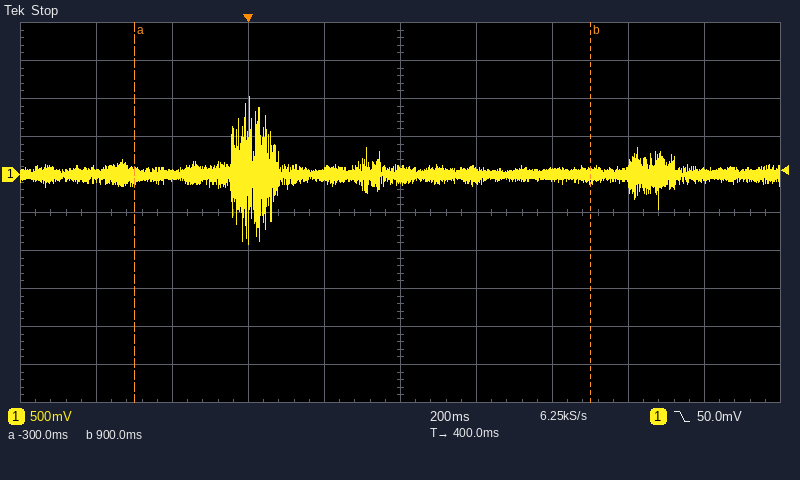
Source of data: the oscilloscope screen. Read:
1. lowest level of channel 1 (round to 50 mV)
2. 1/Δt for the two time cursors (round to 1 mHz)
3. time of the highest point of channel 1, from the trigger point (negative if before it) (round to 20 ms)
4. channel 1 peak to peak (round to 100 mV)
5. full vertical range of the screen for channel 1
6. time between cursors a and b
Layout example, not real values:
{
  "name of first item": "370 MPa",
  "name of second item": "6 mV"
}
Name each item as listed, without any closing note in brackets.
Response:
{
  "lowest level of channel 1": "-900 mV",
  "1/Δt for the two time cursors": "833 mHz",
  "time of the highest point of channel 1, from the trigger point (negative if before it)": "0 ms",
  "channel 1 peak to peak": "1.90 V",
  "full vertical range of the screen for channel 1": "5 V",
  "time between cursors a and b": "1.20 s"
}
